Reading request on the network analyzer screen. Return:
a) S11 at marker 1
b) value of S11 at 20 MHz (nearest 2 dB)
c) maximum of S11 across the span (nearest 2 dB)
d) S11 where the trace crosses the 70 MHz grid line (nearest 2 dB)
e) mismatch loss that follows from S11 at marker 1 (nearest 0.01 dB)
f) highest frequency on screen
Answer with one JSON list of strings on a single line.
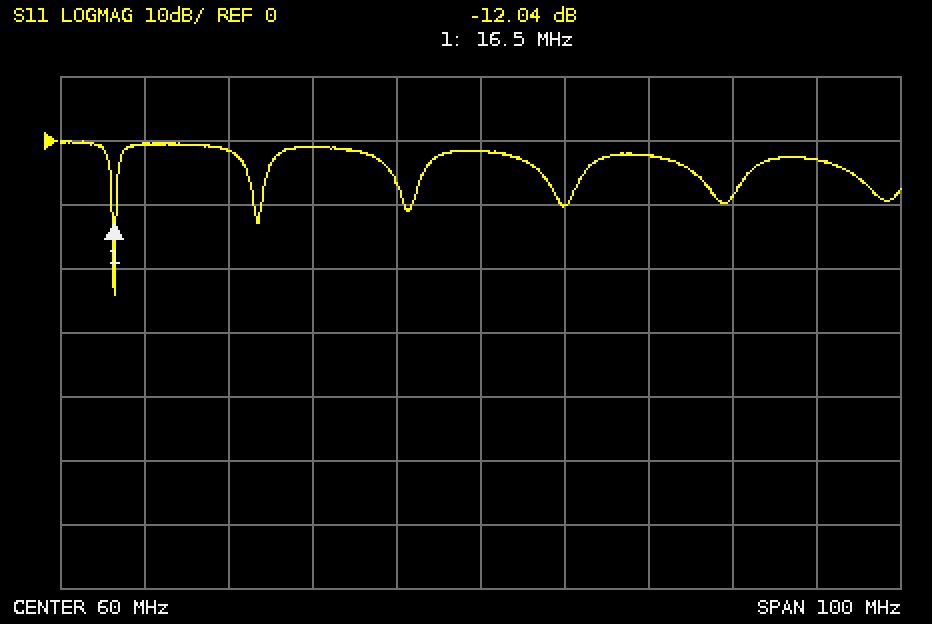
["-12.04 dB", "0 dB", "0 dB", "-10 dB", "0.28 dB", "110 MHz"]
